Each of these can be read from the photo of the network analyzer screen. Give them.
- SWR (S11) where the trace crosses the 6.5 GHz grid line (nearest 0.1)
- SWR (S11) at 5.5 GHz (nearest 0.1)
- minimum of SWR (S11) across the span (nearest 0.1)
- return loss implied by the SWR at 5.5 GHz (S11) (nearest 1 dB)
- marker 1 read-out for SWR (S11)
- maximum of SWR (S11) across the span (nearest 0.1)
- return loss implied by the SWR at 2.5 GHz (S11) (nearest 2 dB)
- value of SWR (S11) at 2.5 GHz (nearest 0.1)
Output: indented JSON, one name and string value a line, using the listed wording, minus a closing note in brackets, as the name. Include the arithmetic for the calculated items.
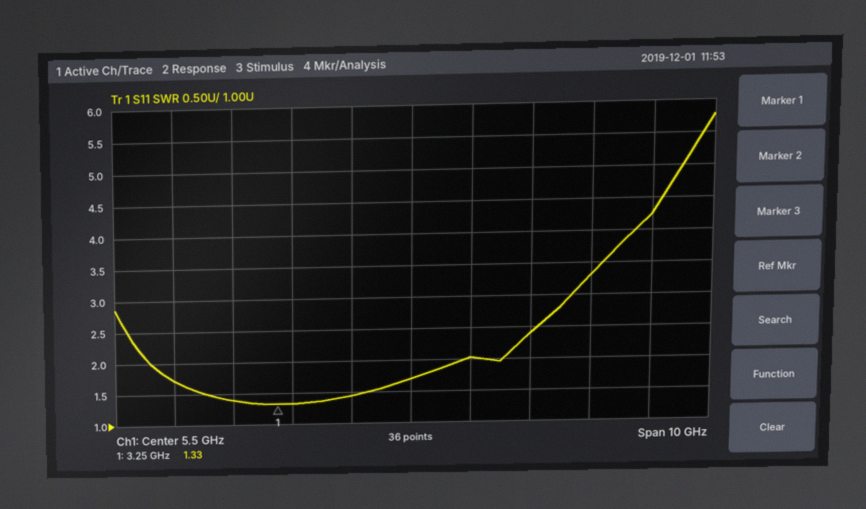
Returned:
{
  "SWR (S11) where the trace crosses the 6.5 GHz grid line": "2.0",
  "SWR (S11) at 5.5 GHz": "1.7",
  "minimum of SWR (S11) across the span": "1.3",
  "return loss implied by the SWR at 5.5 GHz (S11)": "−20 log10((1.7 − 1)/(1.7 + 1)) ≈ 12 dB",
  "marker 1 read-out for SWR": "1.33",
  "maximum of SWR (S11) across the span": "5.8",
  "return loss implied by the SWR at 2.5 GHz (S11)": "−20 log10((1.4 − 1)/(1.4 + 1)) ≈ 16 dB",
  "value of SWR (S11) at 2.5 GHz": "1.4"
}
